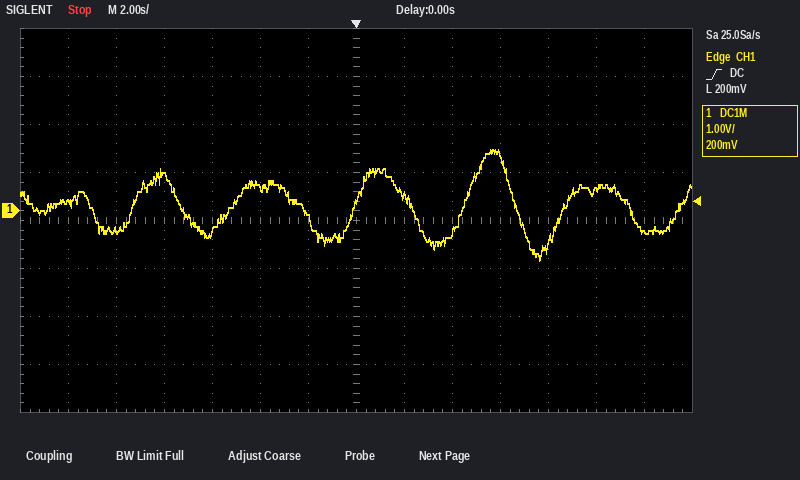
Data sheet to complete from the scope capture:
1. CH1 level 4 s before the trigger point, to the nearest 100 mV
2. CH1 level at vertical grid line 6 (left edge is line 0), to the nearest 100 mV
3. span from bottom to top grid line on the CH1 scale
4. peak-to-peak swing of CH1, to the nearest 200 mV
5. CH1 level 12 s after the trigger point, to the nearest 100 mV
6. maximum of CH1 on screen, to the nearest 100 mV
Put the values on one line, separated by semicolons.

500 mV; -100 mV; 8 V; 2.4 V; -400 mV; 1.3 V
